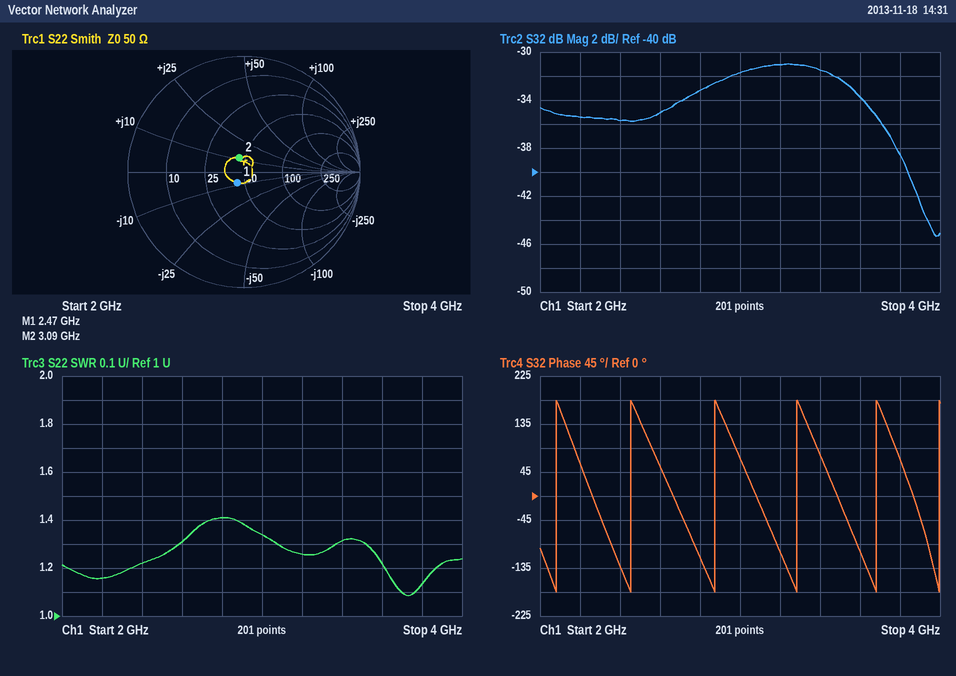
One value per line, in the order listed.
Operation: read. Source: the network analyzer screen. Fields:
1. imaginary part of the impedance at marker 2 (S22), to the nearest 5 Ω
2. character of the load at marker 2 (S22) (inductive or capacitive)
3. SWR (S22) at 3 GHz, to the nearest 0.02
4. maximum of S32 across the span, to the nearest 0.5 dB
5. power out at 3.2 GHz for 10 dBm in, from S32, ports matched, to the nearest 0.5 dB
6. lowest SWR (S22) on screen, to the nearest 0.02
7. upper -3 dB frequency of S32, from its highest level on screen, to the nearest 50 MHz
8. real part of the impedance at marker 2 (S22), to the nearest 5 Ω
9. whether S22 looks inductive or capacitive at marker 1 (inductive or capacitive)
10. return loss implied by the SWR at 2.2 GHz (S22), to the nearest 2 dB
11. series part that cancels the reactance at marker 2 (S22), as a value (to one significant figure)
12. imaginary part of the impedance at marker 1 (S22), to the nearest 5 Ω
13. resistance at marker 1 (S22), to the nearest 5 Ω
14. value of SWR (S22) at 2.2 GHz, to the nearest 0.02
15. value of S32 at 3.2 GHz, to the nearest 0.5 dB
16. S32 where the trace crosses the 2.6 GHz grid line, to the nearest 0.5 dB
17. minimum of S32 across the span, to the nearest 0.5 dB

+10 Ω
inductive
1.34
-31.0 dB
-21.0 dBm
1.08
3.60 GHz
45 Ω
capacitive
22 dB
5 pF
-10 Ω
45 Ω
1.16
-31.0 dB
-35.0 dB
-45.5 dB
